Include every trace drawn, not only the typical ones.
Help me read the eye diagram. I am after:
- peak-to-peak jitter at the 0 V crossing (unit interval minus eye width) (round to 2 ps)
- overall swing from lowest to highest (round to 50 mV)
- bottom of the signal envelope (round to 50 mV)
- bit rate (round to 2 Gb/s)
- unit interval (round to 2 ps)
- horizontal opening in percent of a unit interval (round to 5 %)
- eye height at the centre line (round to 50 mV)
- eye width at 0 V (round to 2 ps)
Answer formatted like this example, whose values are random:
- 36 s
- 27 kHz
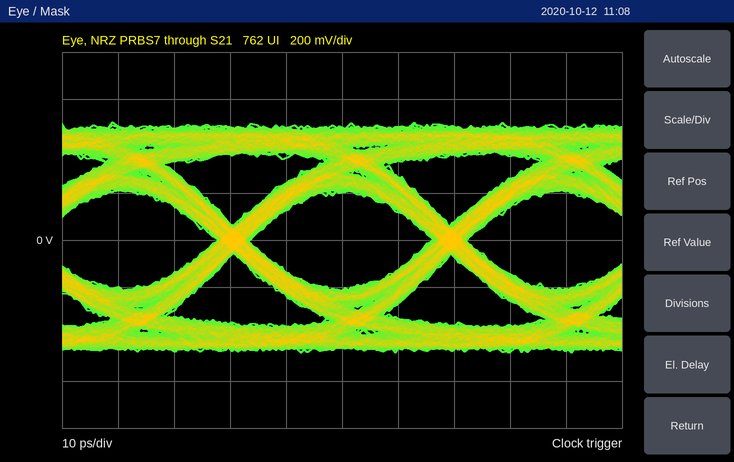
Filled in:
- 6 ps
- 1.00 V
- -500 mV
- 26 Gb/s
- 38 ps
- 85 %
- 400 mV
- 32 ps
